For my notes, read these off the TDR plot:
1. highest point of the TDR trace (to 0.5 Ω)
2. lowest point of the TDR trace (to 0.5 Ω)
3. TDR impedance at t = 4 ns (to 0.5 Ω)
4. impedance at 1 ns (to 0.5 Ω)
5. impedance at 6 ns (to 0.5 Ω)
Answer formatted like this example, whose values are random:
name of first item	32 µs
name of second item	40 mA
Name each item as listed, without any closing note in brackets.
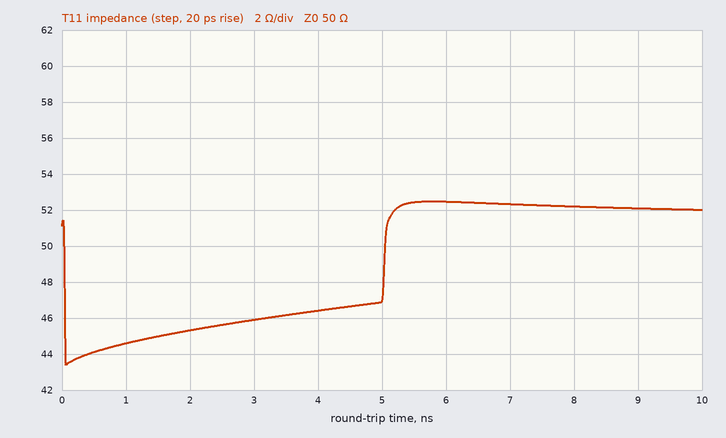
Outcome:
highest point of the TDR trace	52.5 Ω
lowest point of the TDR trace	43.5 Ω
TDR impedance at t = 4 ns	46.5 Ω
impedance at 1 ns	44.5 Ω
impedance at 6 ns	52.5 Ω
